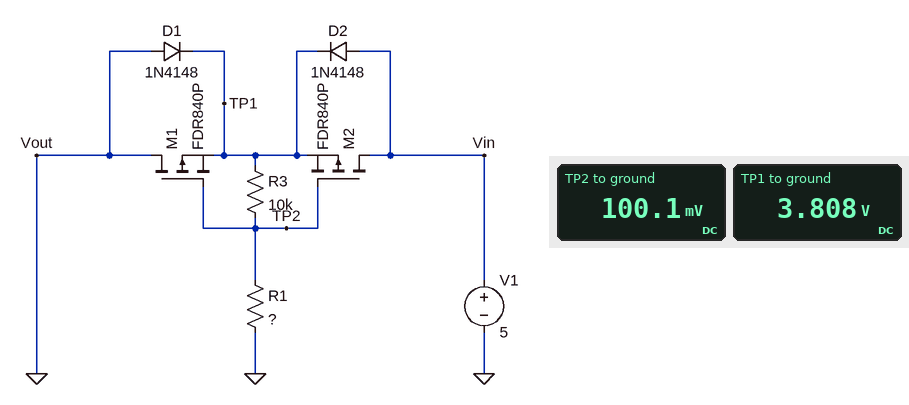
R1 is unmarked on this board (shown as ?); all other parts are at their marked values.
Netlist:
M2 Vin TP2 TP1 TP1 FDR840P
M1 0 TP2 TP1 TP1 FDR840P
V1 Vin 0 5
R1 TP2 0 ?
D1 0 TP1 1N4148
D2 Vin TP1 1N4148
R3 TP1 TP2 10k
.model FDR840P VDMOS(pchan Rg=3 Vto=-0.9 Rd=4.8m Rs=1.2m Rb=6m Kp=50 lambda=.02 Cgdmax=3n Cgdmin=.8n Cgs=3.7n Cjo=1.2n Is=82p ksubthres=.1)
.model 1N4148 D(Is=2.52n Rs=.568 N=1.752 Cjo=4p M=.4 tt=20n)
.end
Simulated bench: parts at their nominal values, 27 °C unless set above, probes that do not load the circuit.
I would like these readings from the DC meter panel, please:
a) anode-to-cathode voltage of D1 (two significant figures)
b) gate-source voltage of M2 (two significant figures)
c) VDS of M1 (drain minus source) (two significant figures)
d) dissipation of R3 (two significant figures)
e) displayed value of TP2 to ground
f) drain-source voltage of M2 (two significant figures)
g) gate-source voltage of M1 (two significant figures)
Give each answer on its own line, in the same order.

-3.8 V
-3.7 V
-3.8 V
1.4 mW
100.1 mV
1.2 V
-3.7 V
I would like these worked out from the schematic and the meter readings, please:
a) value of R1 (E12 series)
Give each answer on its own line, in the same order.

270 Ω
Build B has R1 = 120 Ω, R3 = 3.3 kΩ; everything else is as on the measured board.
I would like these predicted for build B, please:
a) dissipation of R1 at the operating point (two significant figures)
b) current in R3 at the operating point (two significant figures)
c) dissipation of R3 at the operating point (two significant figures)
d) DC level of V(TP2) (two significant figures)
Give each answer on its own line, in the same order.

150 µW
1.1 mA
4.1 mW
130 mV
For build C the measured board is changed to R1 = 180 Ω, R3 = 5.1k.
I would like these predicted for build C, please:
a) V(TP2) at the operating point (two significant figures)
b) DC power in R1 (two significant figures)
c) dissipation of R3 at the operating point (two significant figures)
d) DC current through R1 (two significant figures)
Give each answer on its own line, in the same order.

130 mV
94 µW
2.7 mW
720 µA
